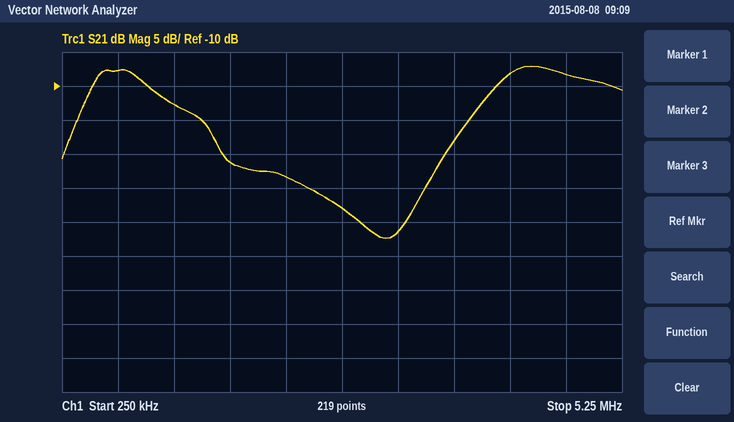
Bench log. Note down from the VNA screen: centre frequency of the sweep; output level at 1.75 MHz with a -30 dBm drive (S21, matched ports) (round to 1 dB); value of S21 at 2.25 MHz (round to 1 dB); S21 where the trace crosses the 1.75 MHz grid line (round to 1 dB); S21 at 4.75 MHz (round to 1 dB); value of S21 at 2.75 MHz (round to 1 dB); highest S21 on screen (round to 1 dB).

2.75 MHz
-51 dBm
-23 dB
-21 dB
-8 dB
-28 dB
-7 dB
